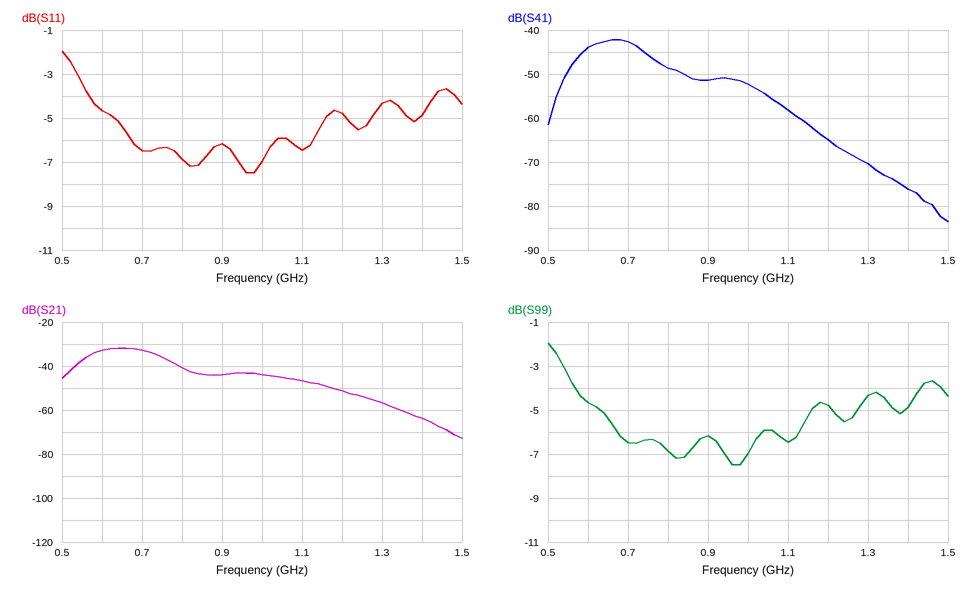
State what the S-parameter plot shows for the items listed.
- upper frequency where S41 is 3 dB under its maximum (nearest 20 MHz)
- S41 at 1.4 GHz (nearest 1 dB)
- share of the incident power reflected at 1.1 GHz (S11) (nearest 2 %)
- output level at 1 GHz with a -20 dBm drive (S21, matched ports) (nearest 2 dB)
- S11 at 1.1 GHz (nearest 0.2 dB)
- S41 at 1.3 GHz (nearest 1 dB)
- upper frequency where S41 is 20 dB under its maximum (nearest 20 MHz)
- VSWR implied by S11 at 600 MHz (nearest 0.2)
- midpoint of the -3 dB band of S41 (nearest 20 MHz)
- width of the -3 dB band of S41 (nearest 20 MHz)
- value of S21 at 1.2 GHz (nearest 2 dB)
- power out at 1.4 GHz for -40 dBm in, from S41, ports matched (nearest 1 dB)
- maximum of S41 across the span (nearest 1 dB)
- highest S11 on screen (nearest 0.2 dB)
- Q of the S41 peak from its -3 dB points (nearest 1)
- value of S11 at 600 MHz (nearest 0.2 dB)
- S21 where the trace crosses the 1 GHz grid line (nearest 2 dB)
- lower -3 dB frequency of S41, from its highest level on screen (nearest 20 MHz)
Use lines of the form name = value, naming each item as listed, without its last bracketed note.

upper frequency where S41 is 3 dB under its maximum = 740 MHz
S41 at 1.4 GHz = -76 dB
share of the incident power reflected at 1.1 GHz (S11) = 22 %
output level at 1 GHz with a -20 dBm drive (S21, matched ports) = -64 dBm
S11 at 1.1 GHz = -6.4 dB
S41 at 1.3 GHz = -70 dB
upper frequency where S41 is 20 dB under its maximum = 1.16 GHz
VSWR implied by S11 at 600 MHz = 3.8
midpoint of the -3 dB band of S41 = 660 MHz
width of the -3 dB band of S41 = 160 MHz
value of S21 at 1.2 GHz = -52 dB
power out at 1.4 GHz for -40 dBm in, from S41, ports matched = -116 dBm
maximum of S41 across the span = -42 dB
highest S11 on screen = -2.0 dB
Q of the S41 peak from its -3 dB points = 4
value of S11 at 600 MHz = -4.6 dB
S21 where the trace crosses the 1 GHz grid line = -44 dB
lower -3 dB frequency of S41, from its highest level on screen = 580 MHz
